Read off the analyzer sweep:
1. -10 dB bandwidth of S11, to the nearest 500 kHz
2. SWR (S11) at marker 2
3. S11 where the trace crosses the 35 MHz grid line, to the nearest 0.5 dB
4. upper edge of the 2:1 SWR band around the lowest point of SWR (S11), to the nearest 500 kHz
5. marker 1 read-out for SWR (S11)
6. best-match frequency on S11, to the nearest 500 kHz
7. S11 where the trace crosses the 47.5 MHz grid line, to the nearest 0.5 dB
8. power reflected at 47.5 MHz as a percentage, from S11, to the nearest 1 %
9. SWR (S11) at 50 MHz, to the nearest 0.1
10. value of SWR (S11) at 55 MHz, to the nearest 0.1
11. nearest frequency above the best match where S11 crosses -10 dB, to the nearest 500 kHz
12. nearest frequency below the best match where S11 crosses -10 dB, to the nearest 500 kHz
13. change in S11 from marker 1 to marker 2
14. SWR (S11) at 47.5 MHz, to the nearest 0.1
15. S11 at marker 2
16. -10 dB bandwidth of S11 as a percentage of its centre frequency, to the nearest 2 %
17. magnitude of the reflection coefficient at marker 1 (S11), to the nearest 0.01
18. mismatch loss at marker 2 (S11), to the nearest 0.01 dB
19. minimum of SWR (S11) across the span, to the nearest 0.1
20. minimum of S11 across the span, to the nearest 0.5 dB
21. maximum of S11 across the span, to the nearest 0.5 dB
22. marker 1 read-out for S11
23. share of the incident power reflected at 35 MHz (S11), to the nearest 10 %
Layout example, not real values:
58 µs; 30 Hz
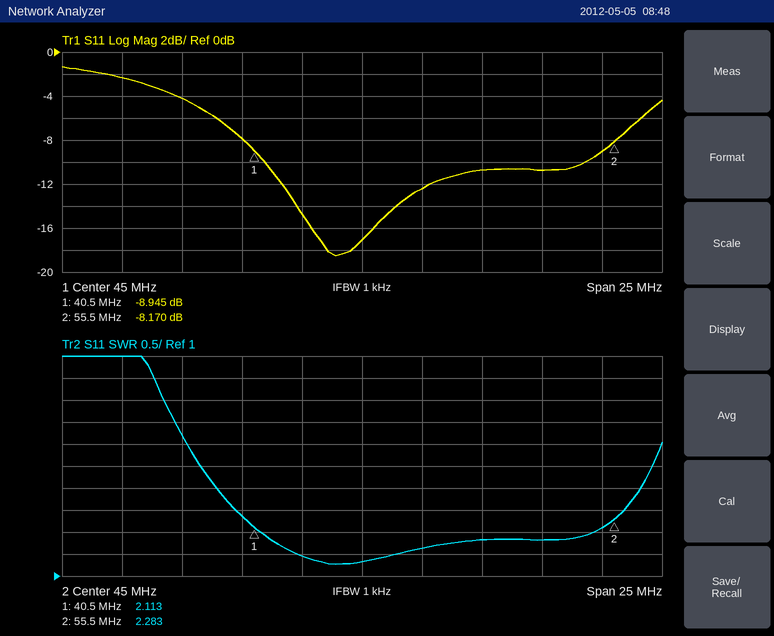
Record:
13.5 MHz; 2.283; -2.5 dB; 54.5 MHz; 2.113; 44.0 MHz; -12.5 dB; 6 %; 1.8; 2.1; 54.5 MHz; 41.0 MHz; 0.775 dB; 1.6; -8.170 dB; 28 %; 0.36; 0.72 dB; 1.3; -18.5 dB; -1.5 dB; -8.945 dB; 60 %
